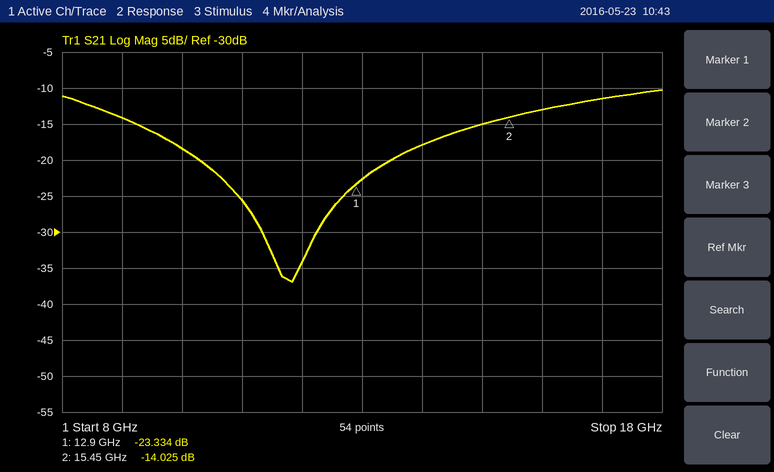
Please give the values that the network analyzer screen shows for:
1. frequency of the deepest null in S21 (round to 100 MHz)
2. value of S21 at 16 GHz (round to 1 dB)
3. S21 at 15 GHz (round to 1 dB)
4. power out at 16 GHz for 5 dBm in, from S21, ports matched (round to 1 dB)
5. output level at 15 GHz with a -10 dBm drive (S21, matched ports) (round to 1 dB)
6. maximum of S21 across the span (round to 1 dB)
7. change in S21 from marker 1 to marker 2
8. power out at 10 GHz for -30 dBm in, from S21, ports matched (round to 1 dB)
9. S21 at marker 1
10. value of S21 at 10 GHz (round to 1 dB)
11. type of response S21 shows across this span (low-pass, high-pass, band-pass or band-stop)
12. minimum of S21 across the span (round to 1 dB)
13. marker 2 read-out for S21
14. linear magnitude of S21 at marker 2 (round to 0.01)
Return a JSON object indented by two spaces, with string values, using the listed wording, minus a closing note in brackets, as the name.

{
  "frequency of the deepest null in S21": "11.8 GHz",
  "value of S21 at 16 GHz": "-13 dB",
  "S21 at 15 GHz": "-15 dB",
  "power out at 16 GHz for 5 dBm in, from S21, ports matched": "-8 dBm",
  "output level at 15 GHz with a -10 dBm drive (S21, matched ports)": "-25 dBm",
  "maximum of S21 across the span": "-10 dB",
  "change in S21 from marker 1 to marker 2": "9.309 dB",
  "power out at 10 GHz for -30 dBm in, from S21, ports matched": "-48 dBm",
  "S21 at marker 1": "-23.334 dB",
  "value of S21 at 10 GHz": "-18 dB",
  "type of response S21 shows across this span": "band-stop",
  "minimum of S21 across the span": "-37 dB",
  "marker 2 read-out for S21": "-14.025 dB",
  "linear magnitude of S21 at marker 2": "0.20"
}
